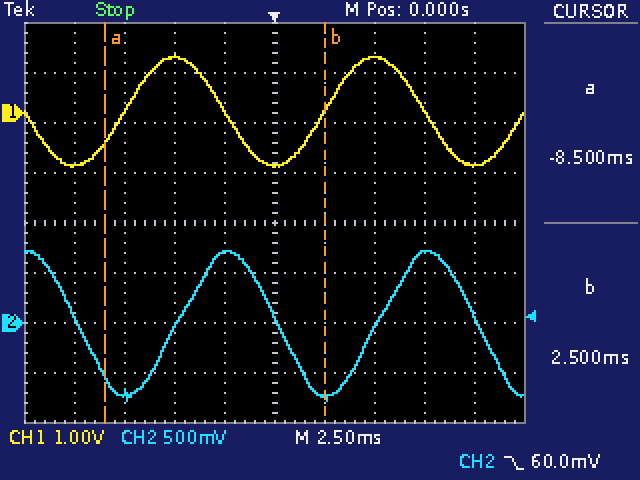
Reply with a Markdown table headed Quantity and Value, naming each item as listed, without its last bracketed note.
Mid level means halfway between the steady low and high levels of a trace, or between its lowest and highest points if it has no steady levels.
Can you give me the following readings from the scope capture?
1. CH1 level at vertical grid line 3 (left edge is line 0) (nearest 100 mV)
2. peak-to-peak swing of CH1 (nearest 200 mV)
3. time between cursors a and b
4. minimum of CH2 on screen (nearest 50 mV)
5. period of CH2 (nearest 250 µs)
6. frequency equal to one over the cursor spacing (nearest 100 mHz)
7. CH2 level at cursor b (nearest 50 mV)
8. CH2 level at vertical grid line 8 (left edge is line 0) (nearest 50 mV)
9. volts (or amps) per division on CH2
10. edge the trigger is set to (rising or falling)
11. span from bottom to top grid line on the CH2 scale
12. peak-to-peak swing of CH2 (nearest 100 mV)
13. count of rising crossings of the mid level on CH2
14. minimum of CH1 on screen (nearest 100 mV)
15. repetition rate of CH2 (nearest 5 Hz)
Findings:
| Quantity | Value |
|---|---|
| CH1 level at vertical grid line 3 (left edge is line 0) | 1.1 V |
| peak-to-peak swing of CH1 | 2.2 V |
| time between cursors a and b | 11.00 ms |
| minimum of CH2 on screen | -800 mV |
| period of CH2 | 10.00 ms |
| frequency equal to one over the cursor spacing | 90.9 Hz |
| CH2 level at cursor b | -750 mV |
| CH2 level at vertical grid line 8 (left edge is line 0) | 700 mV |
| volts (or amps) per division on CH2 | 500 mV |
| edge the trigger is set to | falling |
| span from bottom to top grid line on the CH2 scale | 4 V |
| peak-to-peak swing of CH2 | 1.50 V |
| count of rising crossings of the mid level on CH2 | 2 |
| minimum of CH1 on screen | -1.1 V |
| repetition rate of CH2 | 100 Hz |
